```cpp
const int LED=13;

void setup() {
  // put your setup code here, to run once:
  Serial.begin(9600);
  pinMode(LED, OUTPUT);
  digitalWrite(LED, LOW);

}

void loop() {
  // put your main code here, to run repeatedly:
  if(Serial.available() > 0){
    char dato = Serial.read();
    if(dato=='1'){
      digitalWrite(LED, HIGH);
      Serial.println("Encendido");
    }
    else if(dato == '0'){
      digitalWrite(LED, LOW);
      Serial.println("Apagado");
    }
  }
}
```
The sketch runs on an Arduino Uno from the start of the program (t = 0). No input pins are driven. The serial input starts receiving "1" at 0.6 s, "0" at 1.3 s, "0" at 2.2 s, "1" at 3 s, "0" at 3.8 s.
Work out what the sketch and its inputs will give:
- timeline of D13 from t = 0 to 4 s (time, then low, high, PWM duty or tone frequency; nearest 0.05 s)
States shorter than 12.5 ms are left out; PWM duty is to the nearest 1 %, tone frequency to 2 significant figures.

0 s low; 0.6 s high; 1.3 s low; 3 s high; 3.8 s low
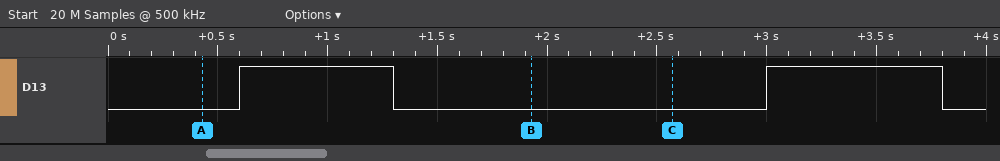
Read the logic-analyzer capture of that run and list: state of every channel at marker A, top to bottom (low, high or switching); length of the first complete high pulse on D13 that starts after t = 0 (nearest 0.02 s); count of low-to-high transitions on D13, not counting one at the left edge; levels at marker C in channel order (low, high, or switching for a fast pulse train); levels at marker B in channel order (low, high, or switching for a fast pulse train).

D13 low
0.70 s
2
D13 low
D13 low
